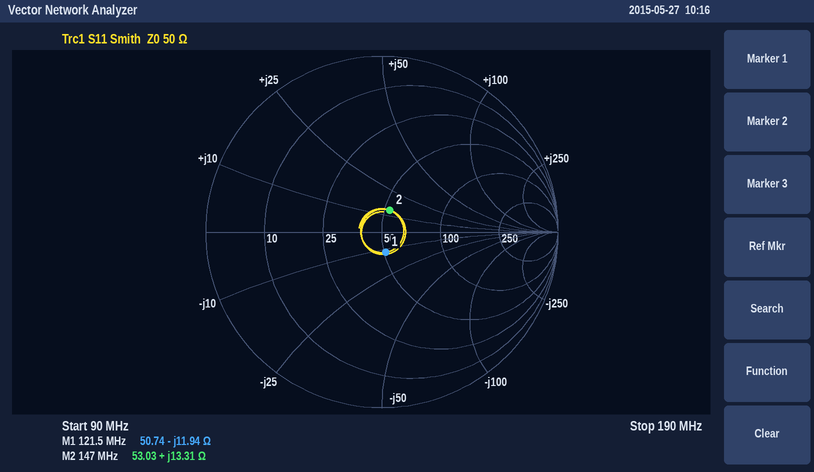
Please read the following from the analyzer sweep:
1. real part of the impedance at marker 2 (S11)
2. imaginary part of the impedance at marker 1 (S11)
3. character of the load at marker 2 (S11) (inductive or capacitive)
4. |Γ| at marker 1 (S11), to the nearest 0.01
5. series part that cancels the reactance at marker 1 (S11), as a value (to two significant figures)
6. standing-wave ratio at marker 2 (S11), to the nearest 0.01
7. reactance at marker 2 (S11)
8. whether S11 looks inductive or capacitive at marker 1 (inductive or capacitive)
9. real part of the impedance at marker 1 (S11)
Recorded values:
53.03 Ω
-11.94 Ω
inductive
0.12
16 nH
1.30
+13.31 Ω
capacitive
50.74 Ω
